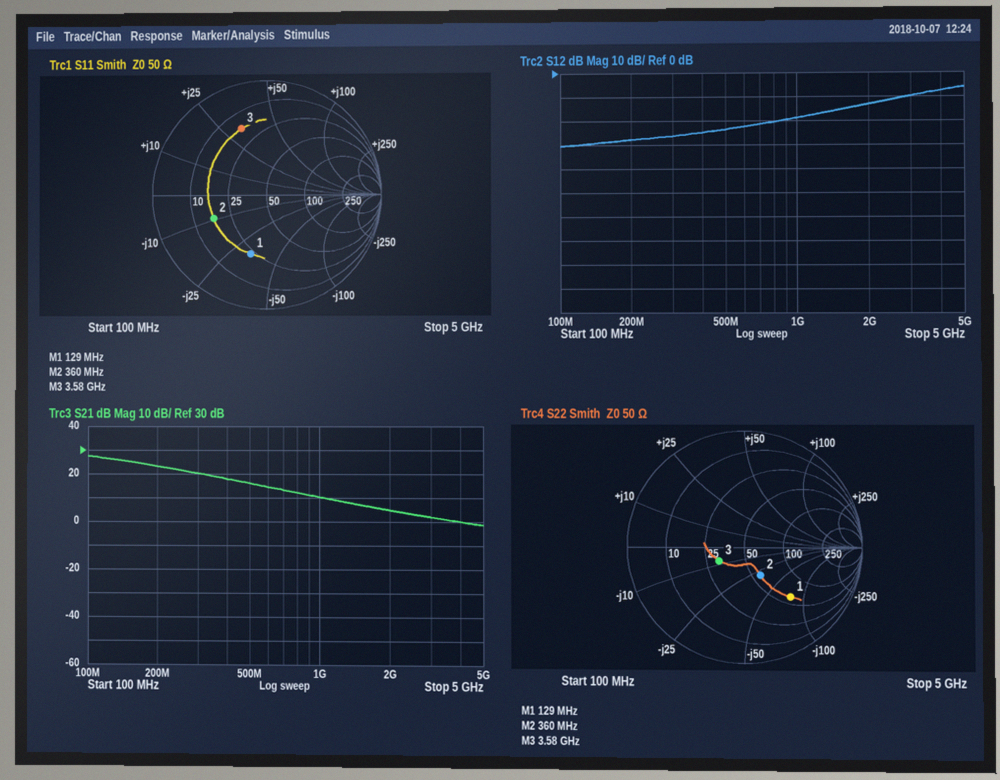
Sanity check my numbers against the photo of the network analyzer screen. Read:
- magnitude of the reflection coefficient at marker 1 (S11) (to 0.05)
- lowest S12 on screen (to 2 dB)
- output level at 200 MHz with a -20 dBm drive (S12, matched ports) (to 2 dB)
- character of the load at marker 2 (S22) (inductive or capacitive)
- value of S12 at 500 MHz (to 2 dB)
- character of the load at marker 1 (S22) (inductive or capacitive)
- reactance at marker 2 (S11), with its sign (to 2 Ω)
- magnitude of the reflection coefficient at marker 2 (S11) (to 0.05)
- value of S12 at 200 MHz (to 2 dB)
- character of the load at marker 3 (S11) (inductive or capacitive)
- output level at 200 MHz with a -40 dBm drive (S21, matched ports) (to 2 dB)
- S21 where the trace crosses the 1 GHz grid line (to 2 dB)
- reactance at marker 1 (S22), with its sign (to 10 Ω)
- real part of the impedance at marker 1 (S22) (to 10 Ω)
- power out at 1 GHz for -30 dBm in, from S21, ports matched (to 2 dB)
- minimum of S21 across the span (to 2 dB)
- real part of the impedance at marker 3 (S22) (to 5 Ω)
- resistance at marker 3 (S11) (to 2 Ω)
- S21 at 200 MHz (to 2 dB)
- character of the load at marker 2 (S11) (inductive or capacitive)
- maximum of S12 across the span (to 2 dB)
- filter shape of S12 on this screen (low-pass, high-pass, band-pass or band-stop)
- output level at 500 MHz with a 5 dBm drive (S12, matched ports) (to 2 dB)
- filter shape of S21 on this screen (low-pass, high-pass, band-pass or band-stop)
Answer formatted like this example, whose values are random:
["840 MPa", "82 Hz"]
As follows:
["0.55", "-30 dB", "-48 dBm", "capacitive", "-24 dB", "capacitive", "-10 Ω", "0.50", "-28 dB", "inductive", "-16 dBm", "10 dB", "-80 Ω", "60 Ω", "-20 dBm", "-2 dB", "30 Ω", "16 Ω", "24 dB", "capacitive", "-6 dB", "high-pass", "-18 dBm", "low-pass"]
